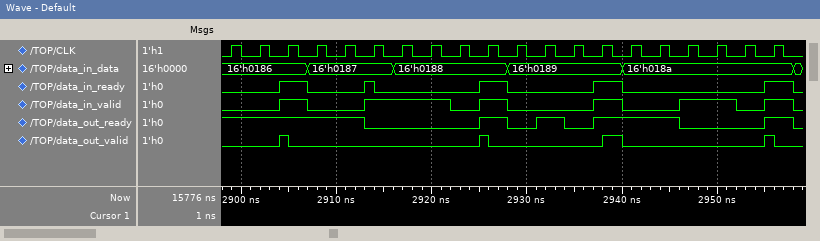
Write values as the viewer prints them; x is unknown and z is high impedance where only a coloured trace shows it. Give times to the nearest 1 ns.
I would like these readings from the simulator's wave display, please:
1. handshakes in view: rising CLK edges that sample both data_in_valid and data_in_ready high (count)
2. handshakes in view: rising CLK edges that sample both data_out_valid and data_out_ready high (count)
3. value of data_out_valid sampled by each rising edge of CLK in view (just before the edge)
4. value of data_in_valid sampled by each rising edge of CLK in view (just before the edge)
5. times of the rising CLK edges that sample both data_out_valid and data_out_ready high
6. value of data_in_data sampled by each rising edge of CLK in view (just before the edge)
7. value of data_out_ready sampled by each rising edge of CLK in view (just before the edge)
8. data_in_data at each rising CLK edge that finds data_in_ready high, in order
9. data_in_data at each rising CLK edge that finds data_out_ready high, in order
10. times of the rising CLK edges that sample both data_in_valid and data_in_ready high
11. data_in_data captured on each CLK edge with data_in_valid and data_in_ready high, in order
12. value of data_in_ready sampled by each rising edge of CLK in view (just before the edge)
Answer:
5
3
0 0 1 0 0 0 0 0 0 1 0 0 0 0 0 0 0 0 0 1
0 0 1 0 0 1 1 1 0 1 0 0 0 1 0 0 1 1 0 1
2905 ns, 2926 ns, 2956 ns
16'h0186, 16'h0186, 16'h0186, 16'h0187, 16'h0187, 16'h0187, 16'h0188, 16'h0188, 16'h0188, 16'h0188, 16'h0189, 16'h0189, 16'h0189, 16'h0189, 16'h018a, 16'h018a, 16'h018a, 16'h018a, 16'h018a, 16'h018a
1 1 1 1 1 0 0 0 0 1 0 1 0 1 1 1 0 0 0 1
16'h0186, 16'h0187, 16'h0188, 16'h0189, 16'h018a
16'h0186, 16'h0186, 16'h0186, 16'h0187, 16'h0187, 16'h0188, 16'h0189, 16'h0189, 16'h018a, 16'h018a, 16'h018a
2905 ns, 2914 ns, 2926 ns, 2938 ns, 2956 ns
16'h0186, 16'h0187, 16'h0188, 16'h0189, 16'h018a
0 0 1 0 0 1 0 0 0 1 0 0 0 1 0 0 0 0 0 1
